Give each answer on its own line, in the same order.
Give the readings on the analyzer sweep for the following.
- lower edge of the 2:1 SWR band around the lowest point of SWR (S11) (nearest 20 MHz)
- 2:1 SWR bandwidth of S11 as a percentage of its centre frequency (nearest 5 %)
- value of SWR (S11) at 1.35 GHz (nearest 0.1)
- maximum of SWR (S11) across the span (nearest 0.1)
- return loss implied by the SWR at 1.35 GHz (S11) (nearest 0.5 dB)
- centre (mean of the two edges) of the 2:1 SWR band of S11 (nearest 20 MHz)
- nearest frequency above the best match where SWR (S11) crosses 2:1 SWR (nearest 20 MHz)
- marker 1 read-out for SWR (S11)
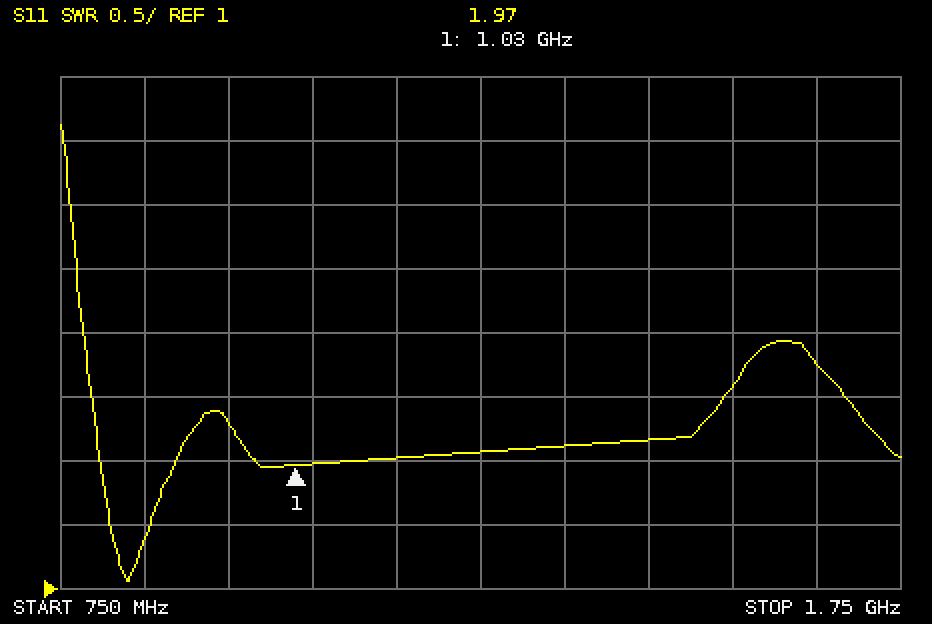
800 MHz
10 %
2.1
4.6
9.0 dB
840 MHz
880 MHz
1.97
